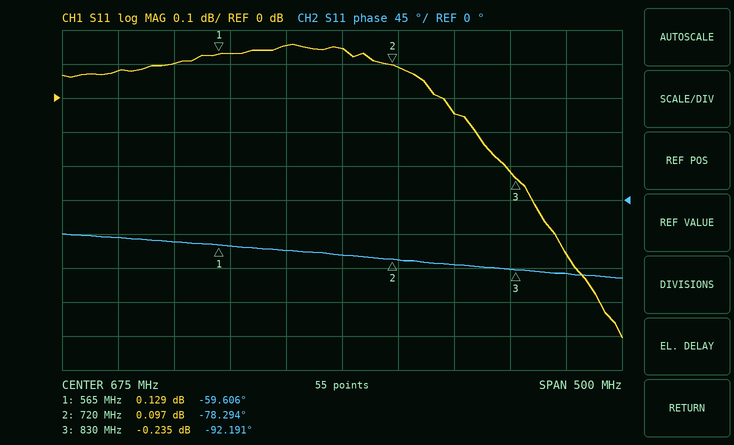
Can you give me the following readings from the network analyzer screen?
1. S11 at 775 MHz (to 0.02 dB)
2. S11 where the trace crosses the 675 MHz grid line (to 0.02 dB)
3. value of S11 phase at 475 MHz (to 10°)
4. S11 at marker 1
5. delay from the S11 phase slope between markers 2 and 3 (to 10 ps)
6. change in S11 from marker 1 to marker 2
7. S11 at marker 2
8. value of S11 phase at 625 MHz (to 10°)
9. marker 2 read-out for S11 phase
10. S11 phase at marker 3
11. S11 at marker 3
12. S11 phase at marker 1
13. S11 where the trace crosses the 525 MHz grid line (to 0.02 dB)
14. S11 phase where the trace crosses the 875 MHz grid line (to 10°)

-0.04 dB
0.14 dB
-50°
0.129 dB
350 ps
-0.032 dB
0.097 dB
-70°
-78.294°
-92.191°
-0.235 dB
-59.606°
0.10 dB
-100°
